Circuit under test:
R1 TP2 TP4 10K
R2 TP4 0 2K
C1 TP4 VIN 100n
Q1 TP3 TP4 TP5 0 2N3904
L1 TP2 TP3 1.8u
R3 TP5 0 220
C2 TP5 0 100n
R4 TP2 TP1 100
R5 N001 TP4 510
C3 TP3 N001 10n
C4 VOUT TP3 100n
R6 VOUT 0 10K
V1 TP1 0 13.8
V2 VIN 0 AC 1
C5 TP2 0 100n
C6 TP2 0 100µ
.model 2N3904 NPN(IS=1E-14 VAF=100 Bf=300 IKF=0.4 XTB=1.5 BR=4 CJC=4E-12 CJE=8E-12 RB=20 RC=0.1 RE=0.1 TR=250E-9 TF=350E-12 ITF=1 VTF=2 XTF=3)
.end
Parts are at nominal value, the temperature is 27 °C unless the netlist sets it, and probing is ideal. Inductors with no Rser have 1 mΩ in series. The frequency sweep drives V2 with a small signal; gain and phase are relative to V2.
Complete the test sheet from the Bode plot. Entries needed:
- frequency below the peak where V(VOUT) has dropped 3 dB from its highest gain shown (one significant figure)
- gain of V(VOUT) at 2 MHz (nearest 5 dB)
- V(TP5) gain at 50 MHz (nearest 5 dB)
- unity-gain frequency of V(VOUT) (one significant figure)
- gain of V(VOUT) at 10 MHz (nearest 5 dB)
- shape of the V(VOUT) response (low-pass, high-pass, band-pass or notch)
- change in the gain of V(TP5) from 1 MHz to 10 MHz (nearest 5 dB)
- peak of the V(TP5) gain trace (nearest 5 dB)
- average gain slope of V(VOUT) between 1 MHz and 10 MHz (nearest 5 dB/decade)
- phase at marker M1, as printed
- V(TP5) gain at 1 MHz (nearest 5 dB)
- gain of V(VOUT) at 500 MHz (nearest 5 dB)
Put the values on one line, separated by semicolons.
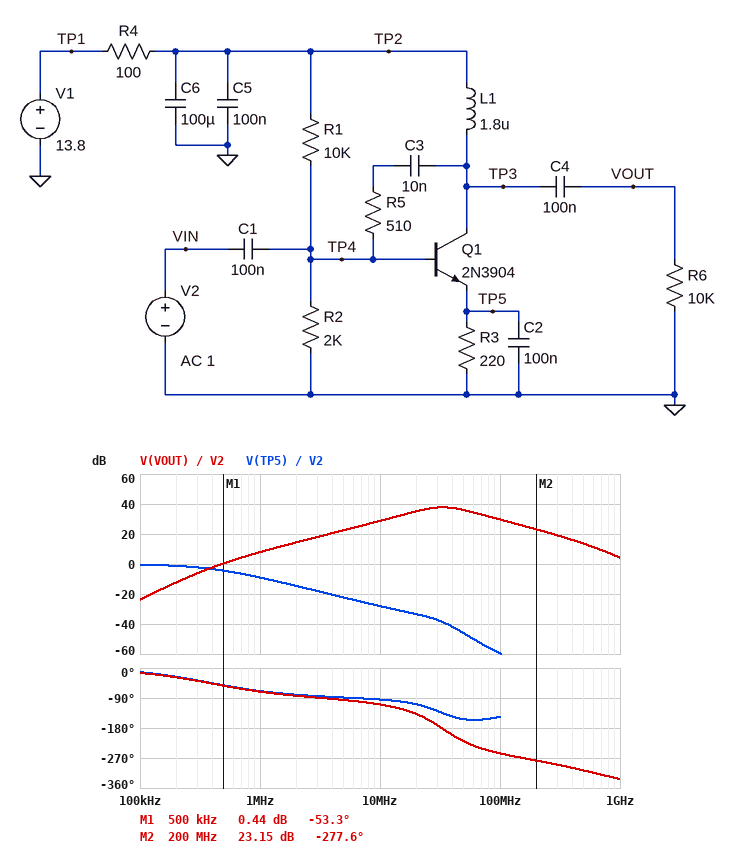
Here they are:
20 MHz; 15 dB; -45 dB; 500 kHz; 30 dB; band-pass; -20 dB; 0 dB; 20 dB/decade; -53.3 deg; -10 dB; 15 dB
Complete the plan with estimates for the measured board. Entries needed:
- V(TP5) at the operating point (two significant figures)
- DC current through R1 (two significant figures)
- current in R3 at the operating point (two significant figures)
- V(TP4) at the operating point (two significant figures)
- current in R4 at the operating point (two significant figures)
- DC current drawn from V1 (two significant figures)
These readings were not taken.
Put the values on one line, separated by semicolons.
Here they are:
1.4 V; 1.1 mA; 6.5 mA; 2.1 V; 7.6 mA; 7.6 mA
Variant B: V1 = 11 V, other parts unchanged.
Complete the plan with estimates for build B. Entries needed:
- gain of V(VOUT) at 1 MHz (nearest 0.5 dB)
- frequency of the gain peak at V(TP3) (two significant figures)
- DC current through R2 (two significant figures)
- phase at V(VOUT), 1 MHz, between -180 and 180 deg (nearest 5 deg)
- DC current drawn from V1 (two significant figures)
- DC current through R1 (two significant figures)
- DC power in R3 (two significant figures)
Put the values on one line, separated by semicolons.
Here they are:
5.5 dB; 37 MHz; 860 µA; -75 deg; 5.5 mA; 870 µA; 4.8 mW
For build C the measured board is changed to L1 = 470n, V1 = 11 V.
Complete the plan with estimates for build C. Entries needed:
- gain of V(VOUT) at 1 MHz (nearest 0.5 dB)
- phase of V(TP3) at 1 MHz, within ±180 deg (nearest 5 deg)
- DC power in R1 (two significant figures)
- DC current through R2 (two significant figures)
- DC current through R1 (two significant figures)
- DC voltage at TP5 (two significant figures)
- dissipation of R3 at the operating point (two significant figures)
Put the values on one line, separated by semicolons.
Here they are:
-6.5 dB; -75 deg; 7.6 mW; 860 µA; 870 µA; 1.0 V; 4.8 mW
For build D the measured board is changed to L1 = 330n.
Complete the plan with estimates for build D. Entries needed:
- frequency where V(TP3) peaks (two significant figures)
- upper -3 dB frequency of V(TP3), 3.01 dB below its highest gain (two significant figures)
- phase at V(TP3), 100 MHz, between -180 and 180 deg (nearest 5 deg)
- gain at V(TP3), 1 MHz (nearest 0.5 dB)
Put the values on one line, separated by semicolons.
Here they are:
81 MHz; 140 MHz; 150 deg; -7.0 dB
